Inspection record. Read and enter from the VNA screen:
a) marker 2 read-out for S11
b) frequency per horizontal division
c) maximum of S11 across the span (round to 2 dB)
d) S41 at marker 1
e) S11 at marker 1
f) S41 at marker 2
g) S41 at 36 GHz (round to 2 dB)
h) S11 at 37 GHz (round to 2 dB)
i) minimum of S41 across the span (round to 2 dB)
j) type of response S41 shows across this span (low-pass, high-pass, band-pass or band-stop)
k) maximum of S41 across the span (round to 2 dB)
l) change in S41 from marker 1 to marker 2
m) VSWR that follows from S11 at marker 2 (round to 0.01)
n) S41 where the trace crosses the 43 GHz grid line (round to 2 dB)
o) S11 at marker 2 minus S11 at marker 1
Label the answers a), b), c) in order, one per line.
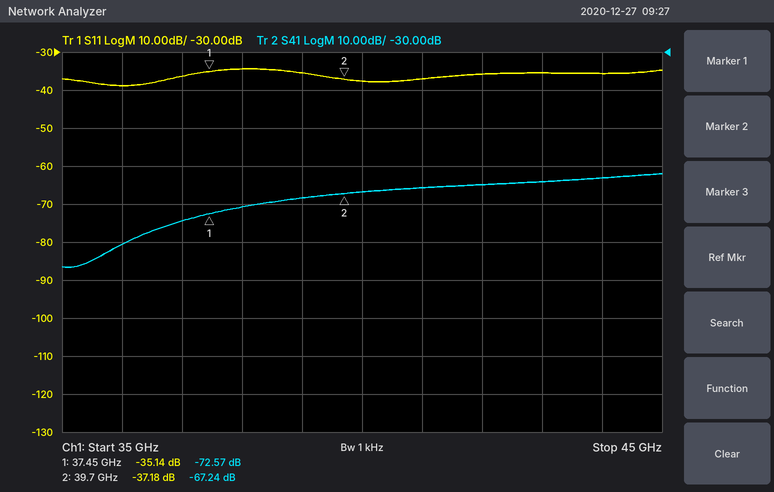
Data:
a) -37.18 dB
b) 1 GHz
c) -34 dB
d) -72.57 dB
e) -35.14 dB
f) -67.24 dB
g) -80 dB
h) -36 dB
i) -86 dB
j) high-pass
k) -62 dB
l) 5.33 dB
m) 1.03
n) -64 dB
o) -2.04 dB
